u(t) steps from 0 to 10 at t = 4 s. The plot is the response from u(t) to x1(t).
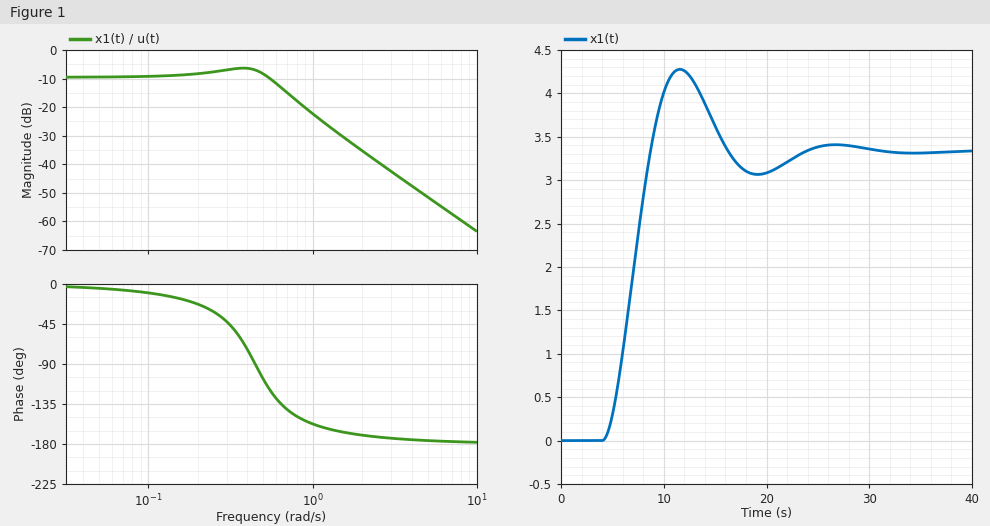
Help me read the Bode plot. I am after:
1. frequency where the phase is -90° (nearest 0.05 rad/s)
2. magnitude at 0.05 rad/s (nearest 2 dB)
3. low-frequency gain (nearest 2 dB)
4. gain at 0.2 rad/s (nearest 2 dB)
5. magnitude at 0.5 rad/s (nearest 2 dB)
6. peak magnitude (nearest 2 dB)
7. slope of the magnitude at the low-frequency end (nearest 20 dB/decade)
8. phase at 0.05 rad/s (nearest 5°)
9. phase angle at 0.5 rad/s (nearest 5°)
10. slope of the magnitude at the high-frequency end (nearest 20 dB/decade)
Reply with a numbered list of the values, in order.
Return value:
1. 0.45 rad/s
2. -10 dB
3. -10 dB
4. -8 dB
5. -8 dB
6. -6 dB
7. 0 dB/decade
8. -5°
9. -105°
10. -40 dB/decade
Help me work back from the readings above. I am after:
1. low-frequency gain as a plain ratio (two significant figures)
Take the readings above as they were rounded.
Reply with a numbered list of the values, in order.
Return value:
1. 0.32
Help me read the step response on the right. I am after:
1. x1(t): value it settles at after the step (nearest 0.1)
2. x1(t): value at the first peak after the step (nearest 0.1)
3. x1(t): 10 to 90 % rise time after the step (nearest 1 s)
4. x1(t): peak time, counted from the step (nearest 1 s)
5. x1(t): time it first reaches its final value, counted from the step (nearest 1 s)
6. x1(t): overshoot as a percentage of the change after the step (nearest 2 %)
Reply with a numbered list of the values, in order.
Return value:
1. 3.3
2. 4.3
3. 3 s
4. 8 s
5. 5 s
6. 28 %
